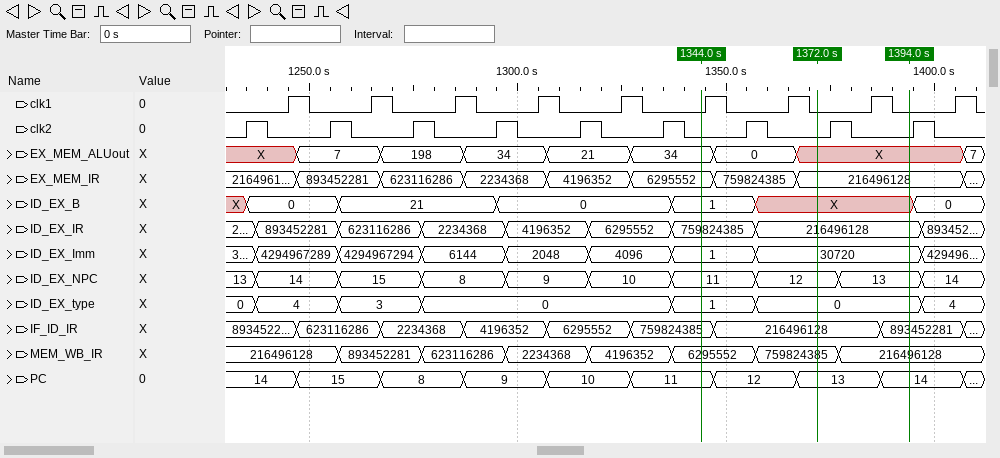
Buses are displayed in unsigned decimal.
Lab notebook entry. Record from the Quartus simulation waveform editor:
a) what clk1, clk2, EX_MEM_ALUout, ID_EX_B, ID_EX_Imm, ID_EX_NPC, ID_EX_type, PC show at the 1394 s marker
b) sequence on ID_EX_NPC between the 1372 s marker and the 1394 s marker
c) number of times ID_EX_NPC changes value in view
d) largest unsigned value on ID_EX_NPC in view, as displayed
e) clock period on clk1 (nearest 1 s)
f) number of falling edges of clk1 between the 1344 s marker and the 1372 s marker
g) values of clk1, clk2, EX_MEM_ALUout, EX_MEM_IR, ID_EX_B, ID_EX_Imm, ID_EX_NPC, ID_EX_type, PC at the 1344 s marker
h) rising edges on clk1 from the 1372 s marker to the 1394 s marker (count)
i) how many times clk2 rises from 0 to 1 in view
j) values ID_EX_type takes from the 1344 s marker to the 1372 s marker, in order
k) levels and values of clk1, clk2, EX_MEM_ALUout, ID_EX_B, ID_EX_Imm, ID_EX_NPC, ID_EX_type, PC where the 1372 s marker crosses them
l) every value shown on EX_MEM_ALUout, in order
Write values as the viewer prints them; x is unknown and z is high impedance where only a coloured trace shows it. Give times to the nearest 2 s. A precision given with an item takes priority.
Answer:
clk1=0, clk2=0, EX_MEM_ALUout=X, ID_EX_B=X, ID_EX_Imm=30720, ID_EX_NPC=13, ID_EX_type=0, PC=14
12, 13
9
15
20 s
2
clk1=0, clk2=0, EX_MEM_ALUout=34, EX_MEM_IR=6295552, ID_EX_B=1, ID_EX_Imm=1, ID_EX_NPC=11, ID_EX_type=1, PC=11
1
9
1, 0
clk1=0, clk2=0, EX_MEM_ALUout=X, ID_EX_B=X, ID_EX_Imm=30720, ID_EX_NPC=12, ID_EX_type=0, PC=13
X, 7, 198, 34, 21, 34, 0, X, 7
